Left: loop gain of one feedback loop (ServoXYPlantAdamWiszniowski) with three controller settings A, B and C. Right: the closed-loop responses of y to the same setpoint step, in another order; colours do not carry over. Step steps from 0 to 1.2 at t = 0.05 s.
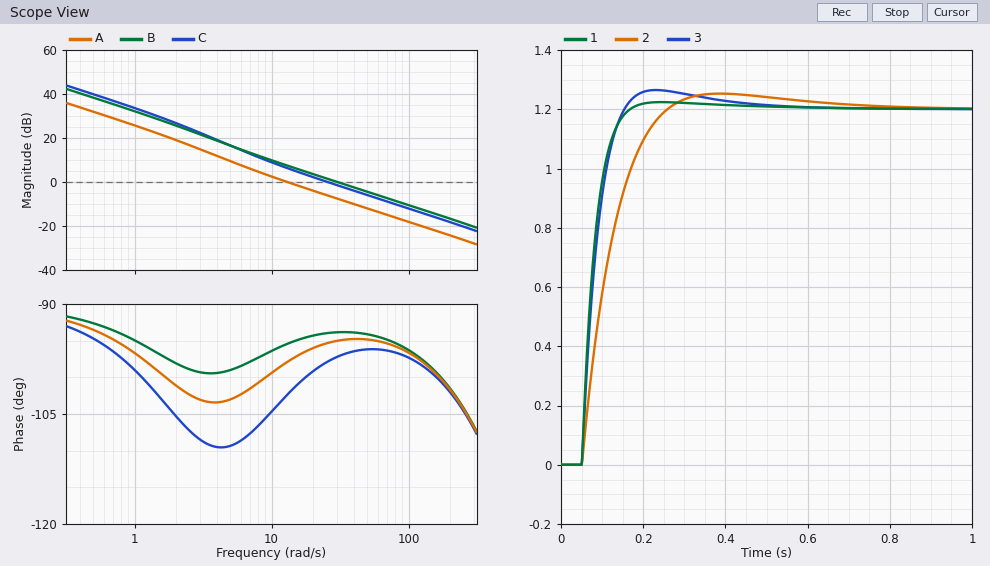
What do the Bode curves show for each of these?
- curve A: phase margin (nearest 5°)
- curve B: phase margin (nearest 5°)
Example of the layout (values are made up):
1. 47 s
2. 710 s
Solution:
1. 80°
2. 85°
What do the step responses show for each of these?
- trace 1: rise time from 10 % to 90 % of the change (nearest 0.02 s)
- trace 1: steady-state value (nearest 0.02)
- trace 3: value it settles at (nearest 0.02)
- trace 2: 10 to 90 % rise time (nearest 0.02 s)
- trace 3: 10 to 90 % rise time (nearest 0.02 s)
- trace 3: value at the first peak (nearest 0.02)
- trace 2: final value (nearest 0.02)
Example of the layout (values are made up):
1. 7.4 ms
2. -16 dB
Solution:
1. 0.06 s
2. 1.20
3. 1.20
4. 0.14 s
5. 0.06 s
6. 1.26
7. 1.20
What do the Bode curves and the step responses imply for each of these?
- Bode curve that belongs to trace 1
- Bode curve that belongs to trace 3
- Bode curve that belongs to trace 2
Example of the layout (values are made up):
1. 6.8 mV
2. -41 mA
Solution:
1. B
2. C
3. A
